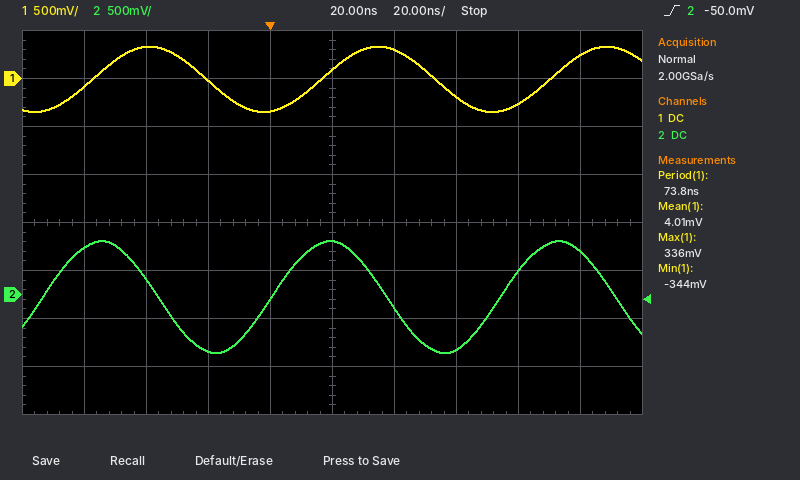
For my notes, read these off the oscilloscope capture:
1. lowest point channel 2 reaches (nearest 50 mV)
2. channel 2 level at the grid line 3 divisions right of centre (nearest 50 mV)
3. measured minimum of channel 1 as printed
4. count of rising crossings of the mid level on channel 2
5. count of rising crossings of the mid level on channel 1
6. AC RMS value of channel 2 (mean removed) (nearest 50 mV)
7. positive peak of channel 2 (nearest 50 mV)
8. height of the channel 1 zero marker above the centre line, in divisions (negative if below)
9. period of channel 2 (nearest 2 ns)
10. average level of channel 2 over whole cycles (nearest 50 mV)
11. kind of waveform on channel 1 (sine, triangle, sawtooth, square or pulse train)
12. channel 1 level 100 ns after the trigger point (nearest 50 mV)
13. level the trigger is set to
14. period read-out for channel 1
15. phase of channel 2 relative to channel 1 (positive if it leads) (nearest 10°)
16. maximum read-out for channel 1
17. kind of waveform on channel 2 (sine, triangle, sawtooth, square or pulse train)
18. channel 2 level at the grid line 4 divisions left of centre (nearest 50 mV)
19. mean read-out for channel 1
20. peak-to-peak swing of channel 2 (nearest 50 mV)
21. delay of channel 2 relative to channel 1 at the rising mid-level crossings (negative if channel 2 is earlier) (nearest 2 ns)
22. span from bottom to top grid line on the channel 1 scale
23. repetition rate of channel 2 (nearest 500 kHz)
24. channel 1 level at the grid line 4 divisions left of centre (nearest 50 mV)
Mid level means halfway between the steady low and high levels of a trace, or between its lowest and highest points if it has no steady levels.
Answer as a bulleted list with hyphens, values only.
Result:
- -600 mV
- 250 mV
- -344 mV
- 3
- 3
- 400 mV
- 550 mV
- +3.0 div
- 74 ns
- 0 mV
- sine
- 250 mV
- -50.0 mV
- 73.8 ns
- +80°
- 336 mV
- sine
- 500 mV
- 4.01 mV
- 1.15 V
- -16 ns
- 4 V
- 13.5 MHz
- -100 mV
